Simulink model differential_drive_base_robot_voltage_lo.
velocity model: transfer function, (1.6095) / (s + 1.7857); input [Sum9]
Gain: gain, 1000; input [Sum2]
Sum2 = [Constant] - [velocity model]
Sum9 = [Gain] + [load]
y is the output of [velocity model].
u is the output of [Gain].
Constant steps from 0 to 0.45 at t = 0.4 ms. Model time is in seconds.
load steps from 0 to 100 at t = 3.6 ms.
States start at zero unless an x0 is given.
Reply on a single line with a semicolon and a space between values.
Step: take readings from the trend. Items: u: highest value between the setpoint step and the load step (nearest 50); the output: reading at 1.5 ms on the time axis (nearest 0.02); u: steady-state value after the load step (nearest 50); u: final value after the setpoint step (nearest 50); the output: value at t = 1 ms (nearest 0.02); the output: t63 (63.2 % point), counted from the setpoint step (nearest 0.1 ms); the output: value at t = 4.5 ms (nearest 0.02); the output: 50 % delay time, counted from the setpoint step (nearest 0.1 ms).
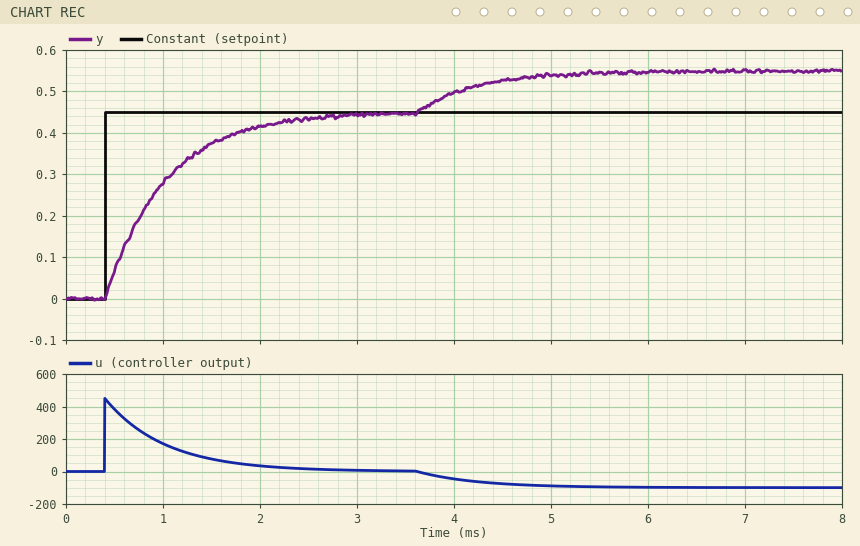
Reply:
450; 0.38; -100; 0; 0.28; 0.6 ms; 0.52; 0.4 ms
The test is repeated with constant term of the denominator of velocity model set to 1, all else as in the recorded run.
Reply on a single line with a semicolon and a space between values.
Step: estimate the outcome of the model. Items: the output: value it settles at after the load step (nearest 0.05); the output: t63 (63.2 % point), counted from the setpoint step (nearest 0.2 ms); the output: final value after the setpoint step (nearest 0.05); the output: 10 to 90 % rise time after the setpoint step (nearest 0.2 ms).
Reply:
0.55; 0.6 ms; 0.45; 1.4 ms
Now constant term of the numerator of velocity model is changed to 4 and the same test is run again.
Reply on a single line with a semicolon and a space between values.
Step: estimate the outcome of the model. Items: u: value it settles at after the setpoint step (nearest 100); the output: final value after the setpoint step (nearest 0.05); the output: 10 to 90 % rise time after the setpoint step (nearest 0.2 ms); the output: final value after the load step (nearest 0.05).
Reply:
0; 0.45; 0.6 ms; 0.55
